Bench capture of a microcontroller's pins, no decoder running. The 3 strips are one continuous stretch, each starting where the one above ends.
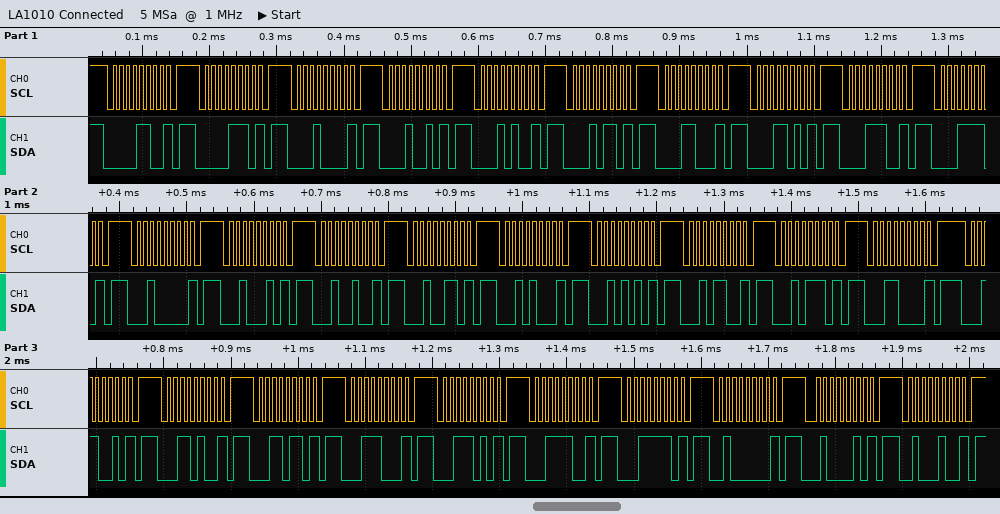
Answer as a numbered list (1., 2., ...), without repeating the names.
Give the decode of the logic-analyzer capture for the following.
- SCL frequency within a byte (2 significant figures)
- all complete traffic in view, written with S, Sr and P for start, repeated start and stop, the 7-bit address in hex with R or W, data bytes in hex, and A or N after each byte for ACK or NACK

1. 100 kHz
2. S 06W N P S 07W N P S 08W N P S 09W N P S 0AW N P S 0BW N P S 0CW N P S 0DW N P S 0EW N P S 0FW N P S 10W N P S 11W N P S 12W N P S 13W N P S 14W N P S 15W N P S 16W N P S 17W N P S 18W N P S 19W N P S 1AW N P S 1BW N P S 1CW N P S 1DW N P S 1EW N P S 1FW N P S 20W N P S 21W N P S 22W N P
